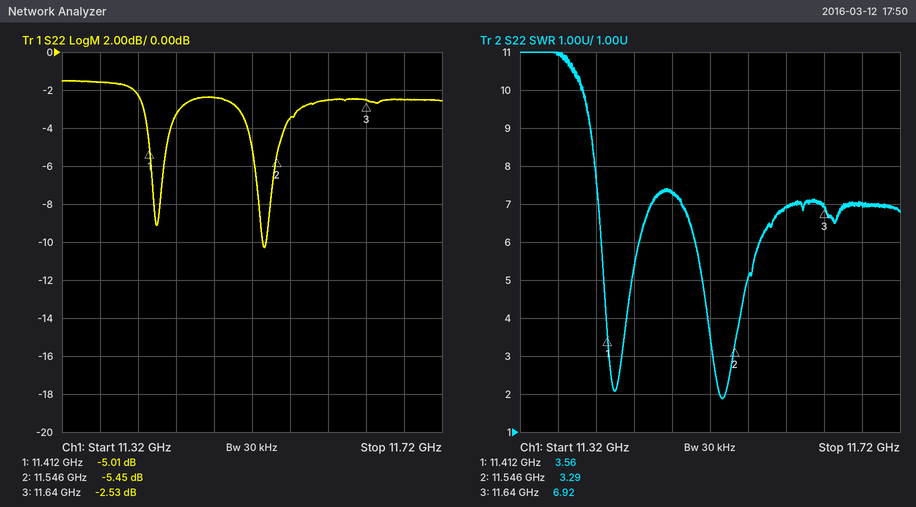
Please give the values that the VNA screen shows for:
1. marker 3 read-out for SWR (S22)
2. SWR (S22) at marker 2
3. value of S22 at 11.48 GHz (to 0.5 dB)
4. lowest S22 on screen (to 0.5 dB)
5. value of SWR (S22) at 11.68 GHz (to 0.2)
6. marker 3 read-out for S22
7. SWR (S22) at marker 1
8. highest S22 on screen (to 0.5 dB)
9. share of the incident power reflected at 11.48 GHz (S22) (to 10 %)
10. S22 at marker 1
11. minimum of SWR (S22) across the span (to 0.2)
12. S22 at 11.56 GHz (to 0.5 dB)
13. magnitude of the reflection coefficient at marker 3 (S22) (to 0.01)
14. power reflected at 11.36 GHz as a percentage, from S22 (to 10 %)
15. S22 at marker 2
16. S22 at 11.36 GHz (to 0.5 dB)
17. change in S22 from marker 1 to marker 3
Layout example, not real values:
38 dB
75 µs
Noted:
6.92
3.29
-2.5 dB
-10.5 dB
7.0
-2.53 dB
3.56
-1.5 dB
60 %
-5.01 dB
1.8
-3.5 dB
0.75
70 %
-5.45 dB
-1.5 dB
2.48 dB
